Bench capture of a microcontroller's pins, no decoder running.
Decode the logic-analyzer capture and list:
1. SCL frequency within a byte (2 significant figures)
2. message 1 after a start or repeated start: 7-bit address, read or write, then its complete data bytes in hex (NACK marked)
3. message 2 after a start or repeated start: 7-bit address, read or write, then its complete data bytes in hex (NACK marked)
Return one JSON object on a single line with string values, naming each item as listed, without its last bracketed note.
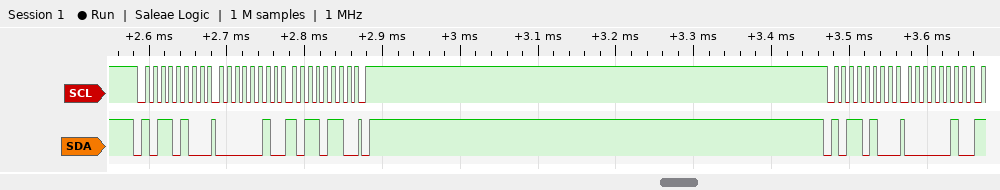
{"SCL frequency within a byte": "100 kHz", "message 1 after a start or repeated start: 7-bit address, read or write, then its complete data bytes in hex": "0x5A write: 02 B6", "message 2 after a start or repeated start: 7-bit address, read or write, then its complete data bytes in hex": "0x5A write: 02"}
